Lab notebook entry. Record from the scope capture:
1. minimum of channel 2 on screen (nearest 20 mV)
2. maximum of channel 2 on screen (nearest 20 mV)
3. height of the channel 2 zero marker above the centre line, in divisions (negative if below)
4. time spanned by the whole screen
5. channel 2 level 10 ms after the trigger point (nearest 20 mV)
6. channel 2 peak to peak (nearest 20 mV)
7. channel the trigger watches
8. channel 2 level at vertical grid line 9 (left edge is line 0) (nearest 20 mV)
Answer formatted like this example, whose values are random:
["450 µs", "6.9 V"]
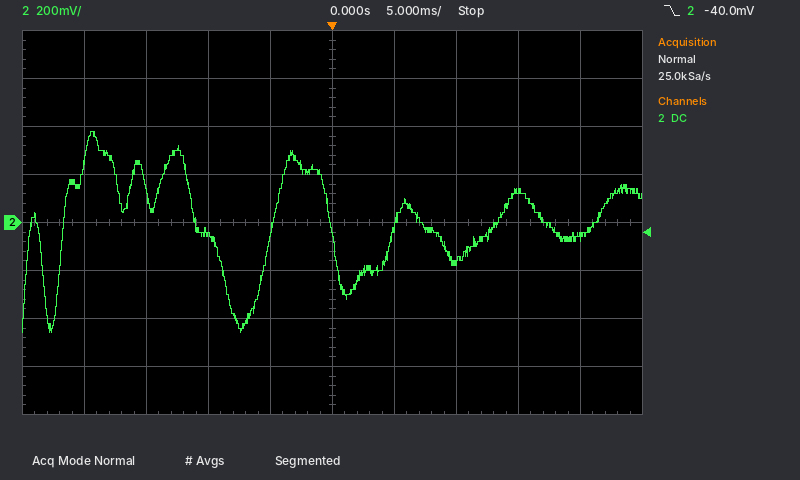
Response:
["-460 mV", "380 mV", "0.0 div", "50 ms", "-160 mV", "840 mV", "channel 2", "-60 mV"]
